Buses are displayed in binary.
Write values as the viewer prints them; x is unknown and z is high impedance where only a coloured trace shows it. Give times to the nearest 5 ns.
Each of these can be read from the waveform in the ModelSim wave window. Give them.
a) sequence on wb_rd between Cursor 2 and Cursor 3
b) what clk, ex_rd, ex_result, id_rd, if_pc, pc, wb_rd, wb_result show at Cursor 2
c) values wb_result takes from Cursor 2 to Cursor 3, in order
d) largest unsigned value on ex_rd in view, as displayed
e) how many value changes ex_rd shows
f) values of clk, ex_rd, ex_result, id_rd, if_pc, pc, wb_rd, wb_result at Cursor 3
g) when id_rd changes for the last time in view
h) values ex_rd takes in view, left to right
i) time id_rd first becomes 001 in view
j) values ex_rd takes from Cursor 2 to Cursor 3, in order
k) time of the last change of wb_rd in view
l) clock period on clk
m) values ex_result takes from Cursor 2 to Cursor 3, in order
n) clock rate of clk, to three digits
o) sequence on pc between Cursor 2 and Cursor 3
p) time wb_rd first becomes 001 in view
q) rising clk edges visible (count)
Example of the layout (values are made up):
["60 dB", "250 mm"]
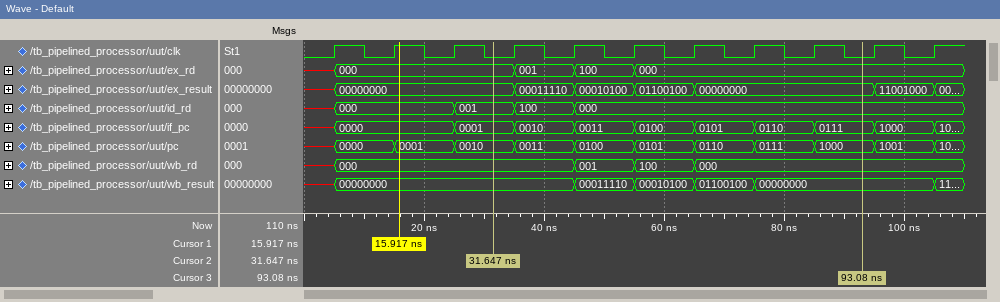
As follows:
["000, 001, 100, 000", "clk=0, ex_rd=000, ex_result=00000000, id_rd=001, if_pc=0001, pc=0010, wb_rd=000, wb_result=00000000", "00000000, 00011110, 00010100, 01100100, 00000000", "100", "4", "clk=0, ex_rd=000, ex_result=00000000, id_rd=000, if_pc=0111, pc=1000, wb_rd=000, wb_result=00000000", "45 ns", "x, 000, 001, 100, 000", "25 ns", "000, 001, 100, 000", "65 ns", "10 ns", "00000000, 00011110, 00010100, 01100100, 00000000", "100 MHz", "0010, 0011, 0100, 0101, 0110, 0111, 1000", "45 ns", "11"]
